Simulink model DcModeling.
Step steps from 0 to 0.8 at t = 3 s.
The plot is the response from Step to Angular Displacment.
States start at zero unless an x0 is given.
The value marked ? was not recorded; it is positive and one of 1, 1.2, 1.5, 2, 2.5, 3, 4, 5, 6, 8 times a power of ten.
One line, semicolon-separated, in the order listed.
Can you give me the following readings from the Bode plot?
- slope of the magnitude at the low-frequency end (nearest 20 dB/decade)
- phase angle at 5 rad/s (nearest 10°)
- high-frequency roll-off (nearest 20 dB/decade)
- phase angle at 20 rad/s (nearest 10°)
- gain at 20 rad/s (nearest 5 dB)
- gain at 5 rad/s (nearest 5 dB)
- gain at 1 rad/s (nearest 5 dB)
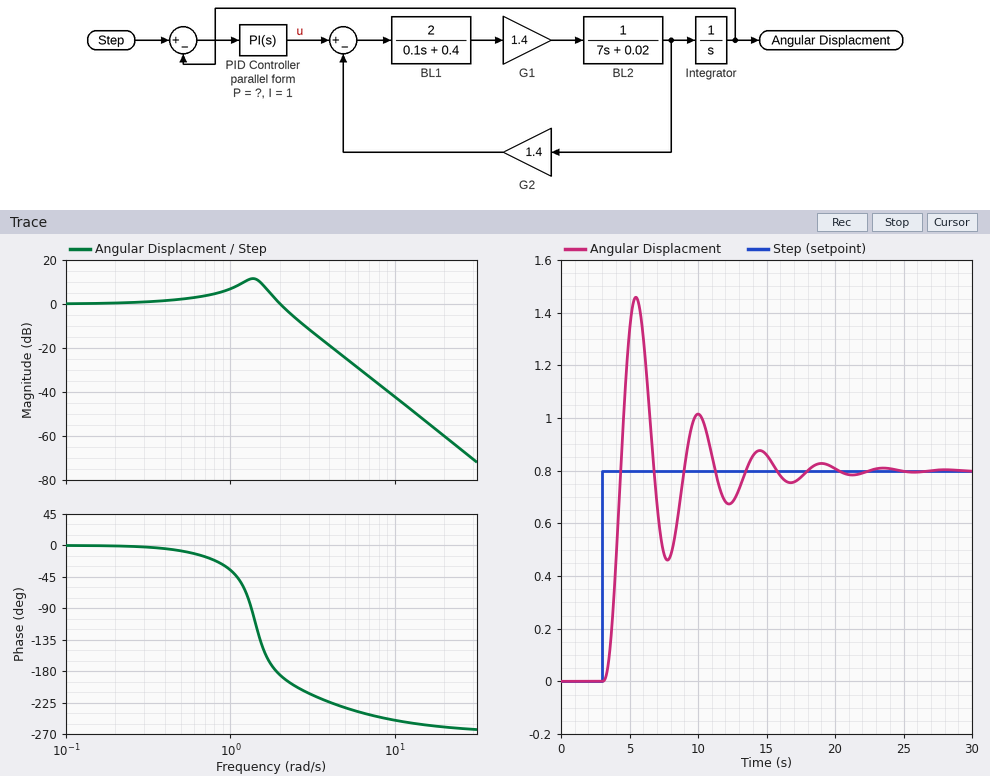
0 dB/decade; -230°; -60 dB/decade; -260°; -60 dB; -25 dB; 5 dB
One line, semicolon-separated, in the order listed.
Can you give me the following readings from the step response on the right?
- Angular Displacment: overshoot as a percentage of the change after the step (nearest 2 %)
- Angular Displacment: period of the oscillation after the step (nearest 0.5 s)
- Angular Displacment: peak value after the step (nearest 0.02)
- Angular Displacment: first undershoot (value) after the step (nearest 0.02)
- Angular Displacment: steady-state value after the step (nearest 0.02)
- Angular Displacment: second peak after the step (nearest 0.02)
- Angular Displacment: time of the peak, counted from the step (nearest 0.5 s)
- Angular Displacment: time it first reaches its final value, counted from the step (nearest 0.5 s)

82 %; 4.5 s; 1.46; 0.46; 0.80; 1.02; 2.5 s; 1.5 s
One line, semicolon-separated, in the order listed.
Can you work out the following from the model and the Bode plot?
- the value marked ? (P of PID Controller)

2
